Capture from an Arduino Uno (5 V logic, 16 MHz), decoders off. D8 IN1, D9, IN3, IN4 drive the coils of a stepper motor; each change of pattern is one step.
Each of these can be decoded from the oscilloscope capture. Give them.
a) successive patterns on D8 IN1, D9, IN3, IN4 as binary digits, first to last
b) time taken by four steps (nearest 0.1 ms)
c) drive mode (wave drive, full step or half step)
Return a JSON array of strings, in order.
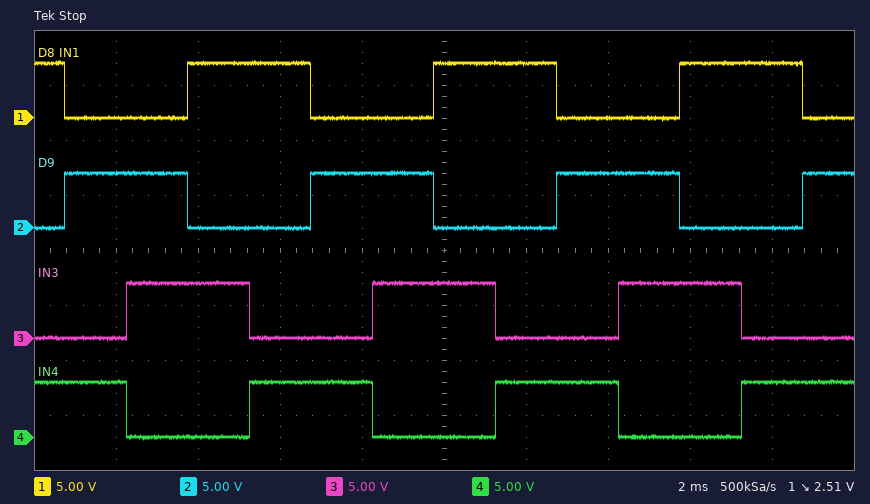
["1001 0101 0110 1010 1001 0101 0110 1010 1001 0101 0110 1010 1001 0101", "6.0 ms", "full step"]
